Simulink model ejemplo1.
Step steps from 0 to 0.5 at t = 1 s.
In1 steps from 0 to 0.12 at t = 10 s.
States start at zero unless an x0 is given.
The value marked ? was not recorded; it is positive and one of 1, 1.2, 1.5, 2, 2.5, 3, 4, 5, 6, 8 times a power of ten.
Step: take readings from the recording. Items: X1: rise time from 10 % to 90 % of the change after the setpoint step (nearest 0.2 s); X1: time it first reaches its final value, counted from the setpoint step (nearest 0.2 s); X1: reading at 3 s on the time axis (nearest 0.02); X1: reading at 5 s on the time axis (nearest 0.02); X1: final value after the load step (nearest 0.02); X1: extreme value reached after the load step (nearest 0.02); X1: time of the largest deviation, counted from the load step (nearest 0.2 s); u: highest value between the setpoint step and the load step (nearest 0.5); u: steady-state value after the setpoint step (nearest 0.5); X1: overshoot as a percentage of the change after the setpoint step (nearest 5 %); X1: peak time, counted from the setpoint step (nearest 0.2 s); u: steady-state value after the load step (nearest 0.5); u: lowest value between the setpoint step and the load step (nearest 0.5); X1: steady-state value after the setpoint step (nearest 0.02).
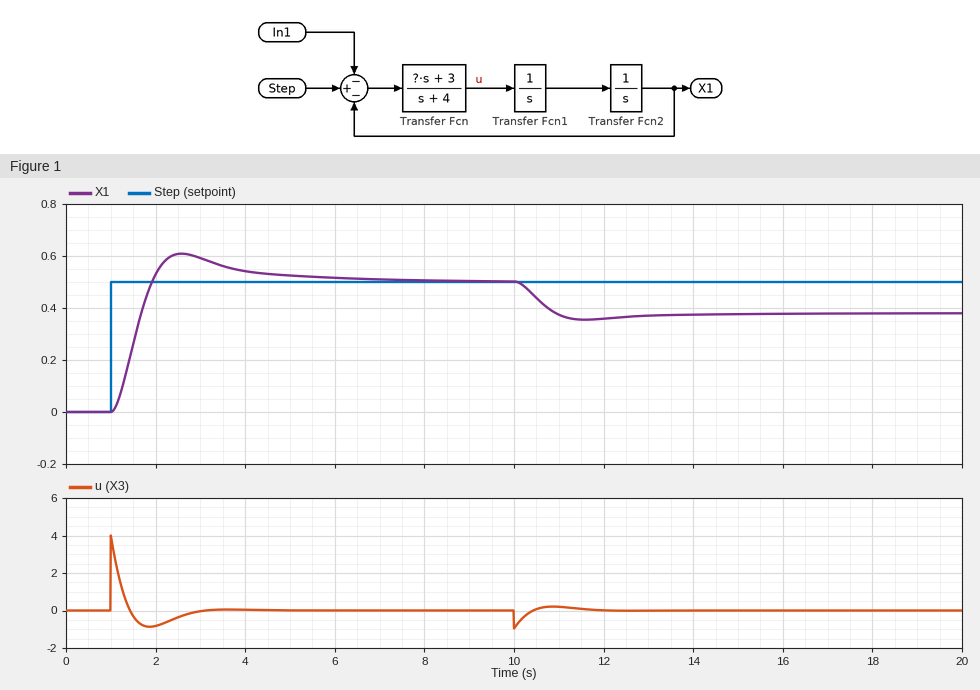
0.6 s
1.0 s
0.60
0.52
0.38
0.36
1.6 s
4.0
0.0
20 %
1.6 s
0.0
-1.0
0.50
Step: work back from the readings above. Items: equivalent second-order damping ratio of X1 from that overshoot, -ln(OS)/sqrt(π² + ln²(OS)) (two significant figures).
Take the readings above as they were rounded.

0.46
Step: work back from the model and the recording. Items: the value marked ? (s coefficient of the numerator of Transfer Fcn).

8
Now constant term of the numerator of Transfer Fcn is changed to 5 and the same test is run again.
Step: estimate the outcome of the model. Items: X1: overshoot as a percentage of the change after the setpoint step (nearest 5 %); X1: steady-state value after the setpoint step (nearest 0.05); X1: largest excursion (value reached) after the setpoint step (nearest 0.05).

30 %
0.50
0.65
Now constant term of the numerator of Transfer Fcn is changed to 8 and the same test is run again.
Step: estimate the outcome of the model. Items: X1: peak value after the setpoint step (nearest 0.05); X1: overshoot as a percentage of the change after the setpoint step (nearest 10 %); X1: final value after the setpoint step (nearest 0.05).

0.70
40 %
0.50
